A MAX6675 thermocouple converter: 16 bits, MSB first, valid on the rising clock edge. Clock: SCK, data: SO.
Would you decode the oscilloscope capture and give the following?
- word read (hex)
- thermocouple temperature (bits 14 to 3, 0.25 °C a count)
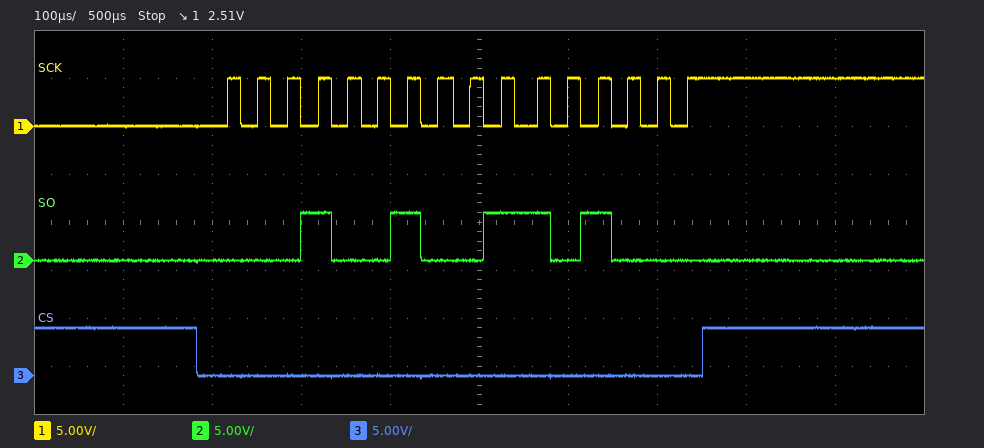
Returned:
0x1268
147.25 °C
